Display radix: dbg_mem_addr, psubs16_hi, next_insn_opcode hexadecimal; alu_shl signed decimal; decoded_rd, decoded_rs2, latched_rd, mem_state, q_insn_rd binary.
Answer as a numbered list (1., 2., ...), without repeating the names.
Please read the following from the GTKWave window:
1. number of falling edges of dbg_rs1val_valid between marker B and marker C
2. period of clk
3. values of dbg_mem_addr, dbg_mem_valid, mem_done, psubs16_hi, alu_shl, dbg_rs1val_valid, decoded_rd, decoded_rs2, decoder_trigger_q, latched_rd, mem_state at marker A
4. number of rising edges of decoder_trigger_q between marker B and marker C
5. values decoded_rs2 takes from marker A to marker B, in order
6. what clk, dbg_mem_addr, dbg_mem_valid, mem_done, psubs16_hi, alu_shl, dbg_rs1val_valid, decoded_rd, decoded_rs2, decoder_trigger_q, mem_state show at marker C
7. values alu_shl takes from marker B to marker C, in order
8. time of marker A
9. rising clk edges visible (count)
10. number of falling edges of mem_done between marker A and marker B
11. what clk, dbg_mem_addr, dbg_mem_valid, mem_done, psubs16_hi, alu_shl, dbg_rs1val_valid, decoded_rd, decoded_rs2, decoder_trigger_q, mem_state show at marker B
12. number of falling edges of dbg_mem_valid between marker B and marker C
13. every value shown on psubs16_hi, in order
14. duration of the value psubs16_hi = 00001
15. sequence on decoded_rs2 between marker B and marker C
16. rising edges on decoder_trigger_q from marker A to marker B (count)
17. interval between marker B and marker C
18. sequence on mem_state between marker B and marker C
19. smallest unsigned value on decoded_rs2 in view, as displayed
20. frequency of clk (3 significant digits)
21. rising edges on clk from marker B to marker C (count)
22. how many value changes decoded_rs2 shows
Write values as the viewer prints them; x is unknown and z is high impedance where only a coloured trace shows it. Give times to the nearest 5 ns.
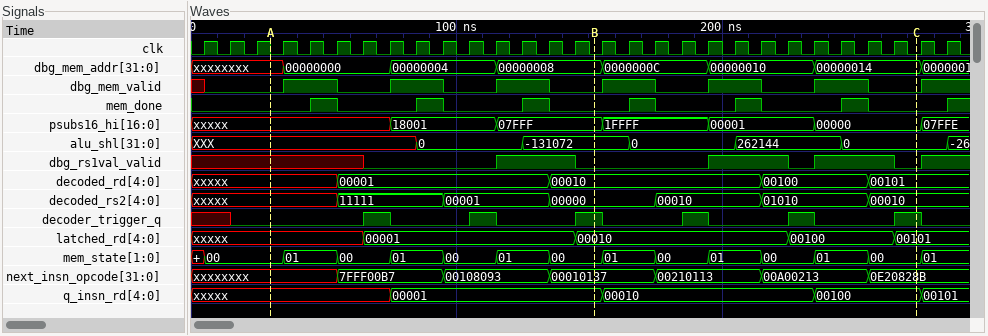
1. 2
2. 10 ns
3. dbg_mem_addr=xxxxxxxx, dbg_mem_valid=0, mem_done=0, psubs16_hi=xxxxx, alu_shl=XXX, dbg_rs1val_valid=x, decoded_rd=xxxxx, decoded_rs2=xxxxx, decoder_trigger_q=0, latched_rd=xxxxx, mem_state=00
4. 3
5. xxxxx, 11111, 00001, 00000
6. clk=0, dbg_mem_addr=00000014, dbg_mem_valid=0, mem_done=0, psubs16_hi=00000, alu_shl=0, dbg_rs1val_valid=0, decoded_rd=00101, decoded_rs2=00010, decoder_trigger_q=1, mem_state=00
7. -131072, 0, 262144, 0
8. 30 ns
9. 29
10. 3
11. clk=0, dbg_mem_addr=00000008, dbg_mem_valid=0, mem_done=0, psubs16_hi=07FFF, alu_shl=-131072, dbg_rs1val_valid=0, decoded_rd=00010, decoded_rs2=00000, decoder_trigger_q=1, mem_state=00
12. 3
13. xxxxx, 18001, 07FFF, 1FFFF, 00001, 00000, 07FFE
14. 40 ns
15. 00000, 00010, 01010, 00010
16. 3
17. 120 ns
18. 00, 01, 00, 01, 00, 01, 00
19. 00000
20. 100 MHz
21. 12
22. 6
